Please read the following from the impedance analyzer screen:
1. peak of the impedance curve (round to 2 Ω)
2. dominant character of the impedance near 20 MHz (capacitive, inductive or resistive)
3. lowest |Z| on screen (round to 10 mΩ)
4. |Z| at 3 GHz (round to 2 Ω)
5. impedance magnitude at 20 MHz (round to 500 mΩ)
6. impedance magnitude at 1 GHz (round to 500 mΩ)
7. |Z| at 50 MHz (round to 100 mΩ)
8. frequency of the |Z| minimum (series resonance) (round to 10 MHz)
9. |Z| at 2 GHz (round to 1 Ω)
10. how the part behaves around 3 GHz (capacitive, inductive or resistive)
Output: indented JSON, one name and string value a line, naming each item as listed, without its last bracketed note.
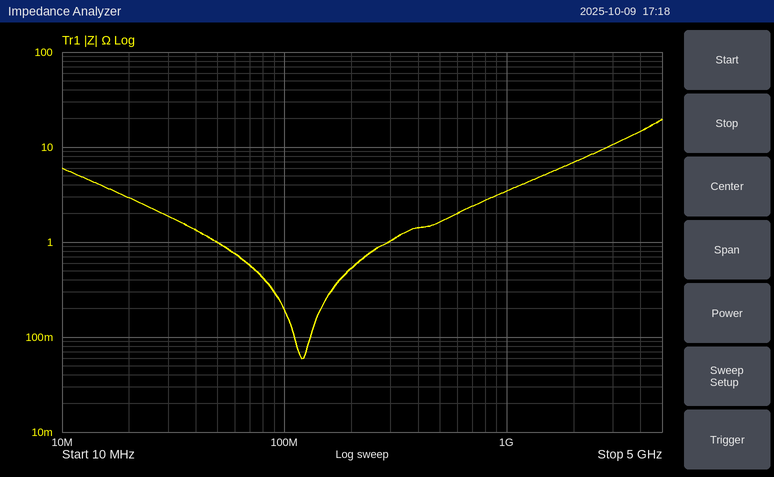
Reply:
{
  "peak of the impedance curve": "20 Ω",
  "dominant character of the impedance near 20 MHz": "capacitive",
  "lowest |Z| on screen": "60 mΩ",
  "|Z| at 3 GHz": "10 Ω",
  "impedance magnitude at 20 MHz": "3.0 Ω",
  "impedance magnitude at 1 GHz": "3.5 Ω",
  "|Z| at 50 MHz": "1.0 Ω",
  "frequency of the |Z| minimum (series resonance)": "120 MHz",
  "|Z| at 2 GHz": "7 Ω",
  "how the part behaves around 3 GHz": "inductive"
}
